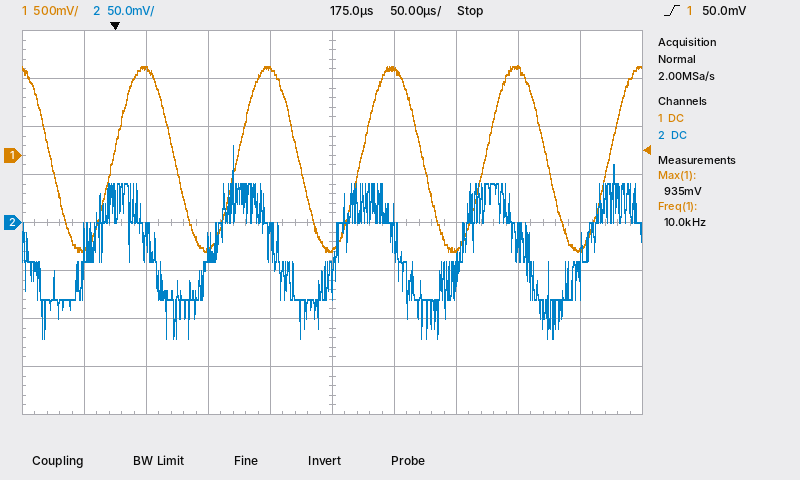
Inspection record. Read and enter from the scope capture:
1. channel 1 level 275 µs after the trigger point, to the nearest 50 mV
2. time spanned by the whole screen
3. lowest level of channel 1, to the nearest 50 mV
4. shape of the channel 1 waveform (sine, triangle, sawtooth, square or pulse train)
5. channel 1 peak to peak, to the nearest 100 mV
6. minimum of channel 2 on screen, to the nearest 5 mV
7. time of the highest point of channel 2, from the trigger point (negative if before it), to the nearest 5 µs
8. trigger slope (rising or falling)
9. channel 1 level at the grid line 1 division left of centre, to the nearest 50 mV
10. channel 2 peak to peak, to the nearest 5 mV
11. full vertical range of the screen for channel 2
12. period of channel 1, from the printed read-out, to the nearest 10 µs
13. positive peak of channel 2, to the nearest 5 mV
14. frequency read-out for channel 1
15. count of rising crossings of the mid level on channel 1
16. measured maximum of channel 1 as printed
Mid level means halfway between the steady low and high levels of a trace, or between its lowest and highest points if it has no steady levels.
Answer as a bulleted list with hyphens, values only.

- -1.00 V
- 500 µs
- -1.00 V
- sine
- 1.90 V
- -120 mV
- +95 µs
- rising
- 900 mV
- 200 mV
- 400 mV
- 100 µs
- 80 mV
- 10.0 kHz
- 5
- 935 mV
